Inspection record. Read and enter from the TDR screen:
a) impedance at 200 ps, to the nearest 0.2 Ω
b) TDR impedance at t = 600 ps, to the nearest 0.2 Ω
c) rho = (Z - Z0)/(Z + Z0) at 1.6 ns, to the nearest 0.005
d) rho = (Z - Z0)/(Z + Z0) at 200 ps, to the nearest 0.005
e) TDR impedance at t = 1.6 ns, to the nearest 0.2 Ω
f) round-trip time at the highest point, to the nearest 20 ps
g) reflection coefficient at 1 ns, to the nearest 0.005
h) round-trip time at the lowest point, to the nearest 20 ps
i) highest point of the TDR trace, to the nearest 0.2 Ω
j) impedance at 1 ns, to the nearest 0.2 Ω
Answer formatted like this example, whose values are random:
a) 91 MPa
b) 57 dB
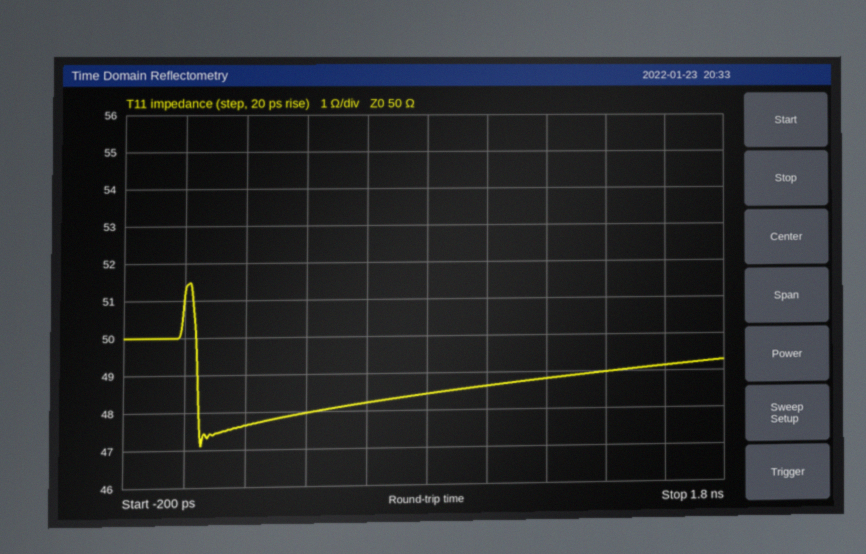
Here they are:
a) 47.6 Ω
b) 48.2 Ω
c) -0.010
d) -0.025
e) 49.2 Ω
f) 20 ps
g) -0.015
h) 60 ps
i) 51.4 Ω
j) 48.6 Ω
